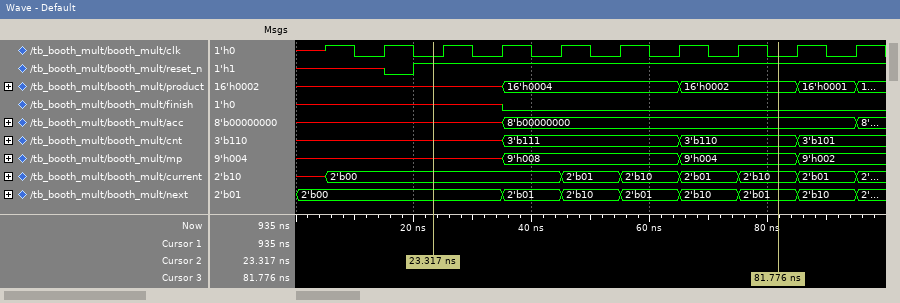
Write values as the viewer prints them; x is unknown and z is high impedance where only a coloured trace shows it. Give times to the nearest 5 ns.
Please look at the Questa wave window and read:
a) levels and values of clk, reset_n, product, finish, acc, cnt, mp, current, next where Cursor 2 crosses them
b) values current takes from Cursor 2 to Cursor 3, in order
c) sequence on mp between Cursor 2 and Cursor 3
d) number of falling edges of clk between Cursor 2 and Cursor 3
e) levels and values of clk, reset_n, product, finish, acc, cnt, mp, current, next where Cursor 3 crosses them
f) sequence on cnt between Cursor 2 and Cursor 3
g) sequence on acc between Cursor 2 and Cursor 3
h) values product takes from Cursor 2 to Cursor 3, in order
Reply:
clk=0, reset_n=1, product=x, finish=x, acc=x, cnt=x, mp=x, current=2'b00, next=2'b00
2'b00, 2'b01, 2'b10, 2'b01, 2'b10
x, 9'h008, 9'h004
6
clk=0, reset_n=1, product=16'h0002, finish=0, acc=8'b00000000, cnt=3'b110, mp=9'h004, current=2'b10, next=2'b01
x, 3'b111, 3'b110
x, 8'b00000000
x, 16'h0004, 16'h0002
